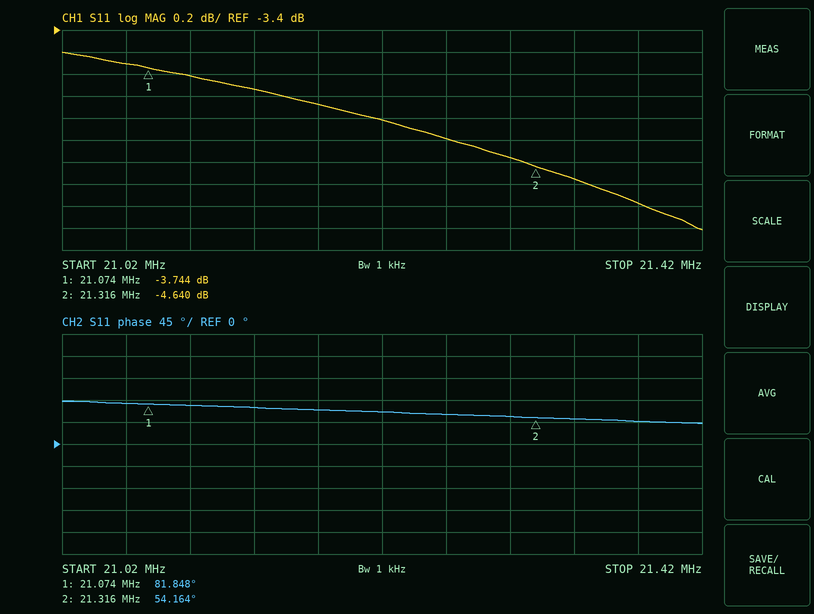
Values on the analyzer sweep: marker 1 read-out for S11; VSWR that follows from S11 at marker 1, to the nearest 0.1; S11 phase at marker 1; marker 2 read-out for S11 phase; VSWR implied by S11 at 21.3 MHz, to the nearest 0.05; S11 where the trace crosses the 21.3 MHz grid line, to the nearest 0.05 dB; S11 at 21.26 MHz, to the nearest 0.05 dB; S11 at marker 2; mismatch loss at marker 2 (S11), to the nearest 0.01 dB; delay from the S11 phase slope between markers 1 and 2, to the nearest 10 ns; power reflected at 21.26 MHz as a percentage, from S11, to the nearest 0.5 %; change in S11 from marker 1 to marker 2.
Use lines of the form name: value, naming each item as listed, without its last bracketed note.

marker 1 read-out for S11: -3.744 dB
VSWR that follows from S11 at marker 1, to the nearest 0.1: 4.7
S11 phase at marker 1: 81.848°
marker 2 read-out for S11 phase: 54.164°
VSWR implied by S11 at 21.3 MHz, to the nearest 0.05: 3.90
S11 where the trace crosses the 21.3 MHz grid line, to the nearest 0.05 dB: -4.55 dB
S11 at 21.26 MHz, to the nearest 0.05 dB: -4.40 dB
S11 at marker 2: -4.640 dB
mismatch loss at marker 2 (S11), to the nearest 0.01 dB: 1.83 dB
delay from the S11 phase slope between markers 1 and 2, to the nearest 10 ns: 320 ns
power reflected at 21.26 MHz as a percentage, from S11, to the nearest 0.5 %: 36.5 %
change in S11 from marker 1 to marker 2: -0.896 dB
